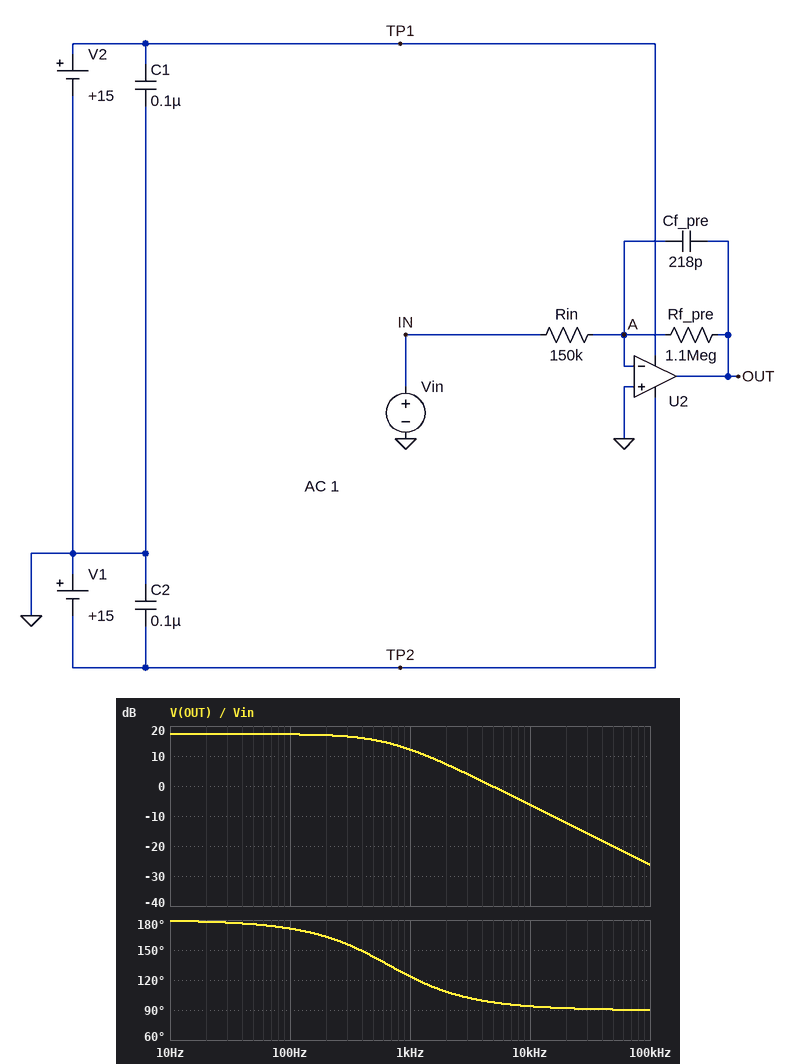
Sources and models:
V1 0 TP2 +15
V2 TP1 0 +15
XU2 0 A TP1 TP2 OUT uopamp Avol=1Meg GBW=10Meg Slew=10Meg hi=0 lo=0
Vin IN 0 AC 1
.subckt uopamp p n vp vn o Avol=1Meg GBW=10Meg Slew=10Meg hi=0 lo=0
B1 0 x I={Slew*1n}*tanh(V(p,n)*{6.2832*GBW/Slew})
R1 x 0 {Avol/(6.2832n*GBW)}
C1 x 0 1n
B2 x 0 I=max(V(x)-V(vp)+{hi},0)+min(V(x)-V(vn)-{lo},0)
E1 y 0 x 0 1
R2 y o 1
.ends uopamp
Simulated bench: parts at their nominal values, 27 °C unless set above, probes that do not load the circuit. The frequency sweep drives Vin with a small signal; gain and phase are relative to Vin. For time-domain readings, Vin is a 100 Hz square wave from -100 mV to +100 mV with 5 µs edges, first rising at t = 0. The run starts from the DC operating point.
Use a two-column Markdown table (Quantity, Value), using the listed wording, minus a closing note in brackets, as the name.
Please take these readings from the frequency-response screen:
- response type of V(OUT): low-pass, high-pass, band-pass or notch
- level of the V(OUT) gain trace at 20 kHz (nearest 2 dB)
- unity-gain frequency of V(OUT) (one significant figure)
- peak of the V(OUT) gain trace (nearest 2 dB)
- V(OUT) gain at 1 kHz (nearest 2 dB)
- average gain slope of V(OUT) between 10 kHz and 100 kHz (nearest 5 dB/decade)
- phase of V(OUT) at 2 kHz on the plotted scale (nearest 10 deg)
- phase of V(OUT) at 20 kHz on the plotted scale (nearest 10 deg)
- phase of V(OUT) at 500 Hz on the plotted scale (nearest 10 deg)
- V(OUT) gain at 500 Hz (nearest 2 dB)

| Quantity | Value |
|---|---|
| response type of V(OUT): low-pass, high-pass, band-pass or notch | low-pass |
| level of the V(OUT) gain trace at 20 kHz | -12 dB |
| unity-gain frequency of V(OUT) | 5 kHz |
| peak of the V(OUT) gain trace | 18 dB |
| V(OUT) gain at 1 kHz | 12 dB |
| average gain slope of V(OUT) between 10 kHz and 100 kHz | -20 dB/decade |
| phase of V(OUT) at 2 kHz on the plotted scale | 110 deg |
| phase of V(OUT) at 20 kHz on the plotted scale | 90 deg |
| phase of V(OUT) at 500 Hz on the plotted scale | 140 deg |
| V(OUT) gain at 500 Hz | 16 dB |
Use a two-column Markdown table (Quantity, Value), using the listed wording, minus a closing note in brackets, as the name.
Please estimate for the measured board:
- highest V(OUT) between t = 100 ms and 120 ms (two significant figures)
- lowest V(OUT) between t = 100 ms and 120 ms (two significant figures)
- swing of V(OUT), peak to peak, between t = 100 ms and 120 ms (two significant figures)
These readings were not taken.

| Quantity | Value |
|---|---|
| highest V(OUT) between t = 100 ms and 120 ms | 730 mV |
| lowest V(OUT) between t = 100 ms and 120 ms | -730 mV |
| swing of V(OUT), peak to peak, between t = 100 ms and 120 ms | 1.5 V |
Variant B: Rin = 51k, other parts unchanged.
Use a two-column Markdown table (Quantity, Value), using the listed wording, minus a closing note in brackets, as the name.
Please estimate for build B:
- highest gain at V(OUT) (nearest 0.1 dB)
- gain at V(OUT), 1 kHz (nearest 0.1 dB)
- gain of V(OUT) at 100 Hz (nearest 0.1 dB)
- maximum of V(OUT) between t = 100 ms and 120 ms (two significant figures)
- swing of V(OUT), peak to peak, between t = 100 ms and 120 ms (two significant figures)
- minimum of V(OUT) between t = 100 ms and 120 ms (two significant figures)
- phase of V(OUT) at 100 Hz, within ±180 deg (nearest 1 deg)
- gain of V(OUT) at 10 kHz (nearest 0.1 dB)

| Quantity | Value |
|---|---|
| highest gain at V(OUT) | 26.7 dB |
| gain at V(OUT), 1 kHz | 21.5 dB |
| gain of V(OUT) at 100 Hz | 26.6 dB |
| maximum of V(OUT) between t = 100 ms and 120 ms | 2.2 V |
| swing of V(OUT), peak to peak, between t = 100 ms and 120 ms | 4.3 V |
| minimum of V(OUT) between t = 100 ms and 120 ms | -2.2 V |
| phase of V(OUT) at 100 Hz, within ±180 deg | 171 deg |
| gain of V(OUT) at 10 kHz | 3.1 dB |
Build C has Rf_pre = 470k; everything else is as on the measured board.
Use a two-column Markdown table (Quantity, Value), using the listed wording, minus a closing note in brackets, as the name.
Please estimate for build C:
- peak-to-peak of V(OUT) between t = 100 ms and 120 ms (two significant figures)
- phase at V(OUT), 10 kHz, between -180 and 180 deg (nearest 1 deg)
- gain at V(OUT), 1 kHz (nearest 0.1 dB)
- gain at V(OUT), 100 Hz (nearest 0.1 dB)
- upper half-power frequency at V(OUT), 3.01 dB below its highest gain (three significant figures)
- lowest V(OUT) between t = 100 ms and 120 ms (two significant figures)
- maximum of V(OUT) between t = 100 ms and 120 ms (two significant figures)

| Quantity | Value |
|---|---|
| peak-to-peak of V(OUT) between t = 100 ms and 120 ms | 630 mV |
| phase at V(OUT), 10 kHz, between -180 and 180 deg | 99 deg |
| gain at V(OUT), 1 kHz | 8.4 dB |
| gain at V(OUT), 100 Hz | 9.9 dB |
| upper half-power frequency at V(OUT), 3.01 dB below its highest gain | 1.55 kHz |
| lowest V(OUT) between t = 100 ms and 120 ms | -310 mV |
| maximum of V(OUT) between t = 100 ms and 120 ms | 310 mV |
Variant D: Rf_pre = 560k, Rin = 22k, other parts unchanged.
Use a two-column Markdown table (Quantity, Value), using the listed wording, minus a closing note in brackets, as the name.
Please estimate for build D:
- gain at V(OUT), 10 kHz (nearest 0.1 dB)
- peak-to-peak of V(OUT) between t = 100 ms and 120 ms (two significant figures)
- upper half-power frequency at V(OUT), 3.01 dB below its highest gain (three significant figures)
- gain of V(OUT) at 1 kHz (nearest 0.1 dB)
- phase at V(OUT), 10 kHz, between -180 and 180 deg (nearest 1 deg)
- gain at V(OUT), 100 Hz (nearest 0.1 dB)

| Quantity | Value |
|---|---|
| gain at V(OUT), 10 kHz | 10.3 dB |
| peak-to-peak of V(OUT) between t = 100 ms and 120 ms | 5.1 V |
| upper half-power frequency at V(OUT), 3.01 dB below its highest gain | 1.30 kHz |
| gain of V(OUT) at 1 kHz | 26.1 dB |
| phase at V(OUT), 10 kHz, between -180 and 180 deg | 97 deg |
| gain at V(OUT), 100 Hz | 28.1 dB |
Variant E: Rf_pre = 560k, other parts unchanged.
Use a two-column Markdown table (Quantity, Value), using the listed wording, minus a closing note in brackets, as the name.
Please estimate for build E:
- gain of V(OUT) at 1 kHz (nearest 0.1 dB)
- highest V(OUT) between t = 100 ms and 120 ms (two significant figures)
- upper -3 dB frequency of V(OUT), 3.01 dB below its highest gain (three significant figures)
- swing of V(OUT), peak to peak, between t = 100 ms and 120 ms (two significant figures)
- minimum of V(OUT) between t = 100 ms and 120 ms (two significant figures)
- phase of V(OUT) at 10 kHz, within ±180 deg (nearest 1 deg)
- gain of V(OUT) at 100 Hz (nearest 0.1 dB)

| Quantity | Value |
|---|---|
| gain of V(OUT) at 1 kHz | 9.4 dB |
| highest V(OUT) between t = 100 ms and 120 ms | 370 mV |
| upper -3 dB frequency of V(OUT), 3.01 dB below its highest gain | 1.30 kHz |
| swing of V(OUT), peak to peak, between t = 100 ms and 120 ms | 750 mV |
| minimum of V(OUT) between t = 100 ms and 120 ms | -370 mV |
| phase of V(OUT) at 10 kHz, within ±180 deg | 97 deg |
| gain of V(OUT) at 100 Hz | 11.4 dB |
